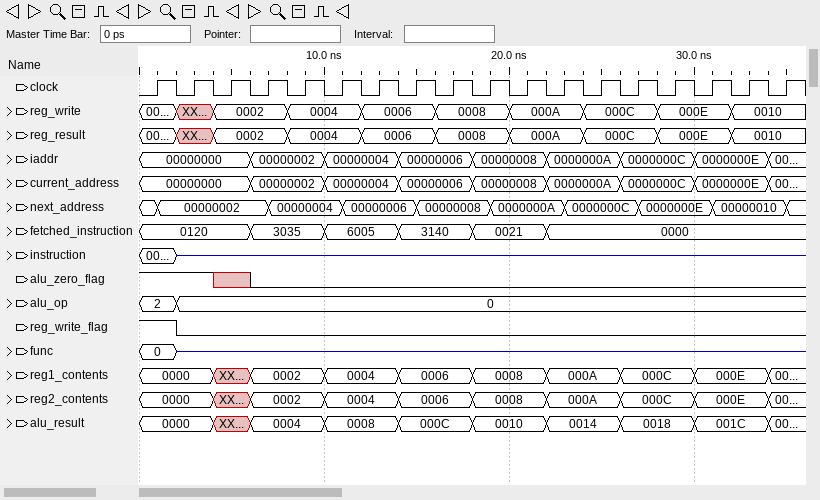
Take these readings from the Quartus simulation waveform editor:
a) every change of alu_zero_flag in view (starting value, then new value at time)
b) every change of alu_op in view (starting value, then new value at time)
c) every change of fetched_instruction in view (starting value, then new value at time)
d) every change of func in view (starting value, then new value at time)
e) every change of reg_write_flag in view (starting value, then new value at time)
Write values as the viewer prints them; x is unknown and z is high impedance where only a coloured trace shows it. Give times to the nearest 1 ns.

1, x at 4 ns, 0 at 6 ns
2, 0 at 2 ns
0120, 3035 at 6 ns, 6005 at 10 ns, 3140 at 14 ns, 0021 at 18 ns, 0000 at 22 ns
0, z at 2 ns
1, 0 at 2 ns
